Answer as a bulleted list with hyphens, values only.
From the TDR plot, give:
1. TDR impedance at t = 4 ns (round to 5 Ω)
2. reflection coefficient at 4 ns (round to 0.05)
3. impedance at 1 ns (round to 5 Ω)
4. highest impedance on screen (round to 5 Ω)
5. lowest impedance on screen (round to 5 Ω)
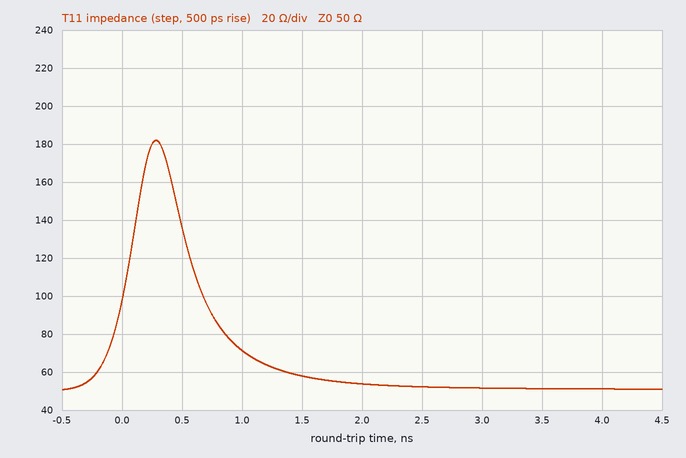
- 50 Ω
- 0.00
- 70 Ω
- 180 Ω
- 50 Ω
